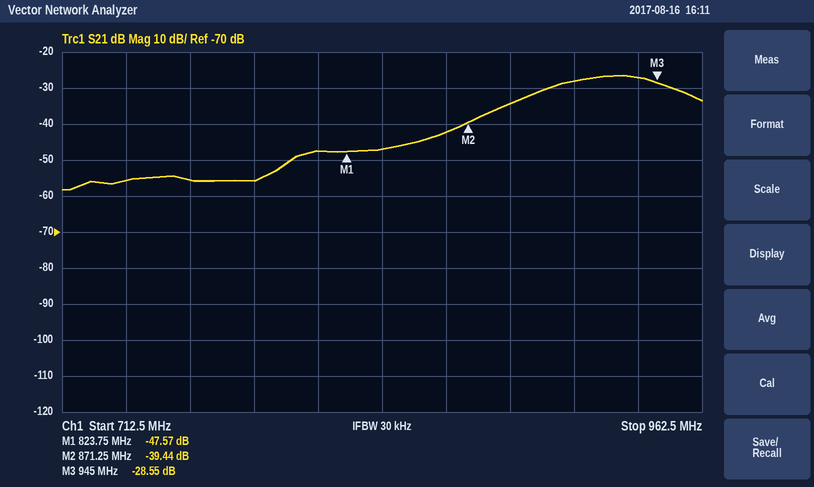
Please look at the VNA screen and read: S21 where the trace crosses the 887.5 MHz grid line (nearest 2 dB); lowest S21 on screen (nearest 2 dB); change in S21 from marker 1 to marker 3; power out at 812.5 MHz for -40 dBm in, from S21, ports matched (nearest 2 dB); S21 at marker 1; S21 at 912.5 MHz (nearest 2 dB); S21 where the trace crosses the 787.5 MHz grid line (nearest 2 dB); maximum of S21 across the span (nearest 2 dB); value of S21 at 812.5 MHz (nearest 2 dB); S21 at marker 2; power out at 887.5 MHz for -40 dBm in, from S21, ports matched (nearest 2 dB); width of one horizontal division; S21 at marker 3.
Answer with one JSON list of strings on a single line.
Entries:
["-34 dB", "-58 dB", "19.02 dB", "-88 dBm", "-47.57 dB", "-28 dB", "-56 dB", "-26 dB", "-48 dB", "-39.44 dB", "-74 dBm", "25 MHz", "-28.55 dB"]
